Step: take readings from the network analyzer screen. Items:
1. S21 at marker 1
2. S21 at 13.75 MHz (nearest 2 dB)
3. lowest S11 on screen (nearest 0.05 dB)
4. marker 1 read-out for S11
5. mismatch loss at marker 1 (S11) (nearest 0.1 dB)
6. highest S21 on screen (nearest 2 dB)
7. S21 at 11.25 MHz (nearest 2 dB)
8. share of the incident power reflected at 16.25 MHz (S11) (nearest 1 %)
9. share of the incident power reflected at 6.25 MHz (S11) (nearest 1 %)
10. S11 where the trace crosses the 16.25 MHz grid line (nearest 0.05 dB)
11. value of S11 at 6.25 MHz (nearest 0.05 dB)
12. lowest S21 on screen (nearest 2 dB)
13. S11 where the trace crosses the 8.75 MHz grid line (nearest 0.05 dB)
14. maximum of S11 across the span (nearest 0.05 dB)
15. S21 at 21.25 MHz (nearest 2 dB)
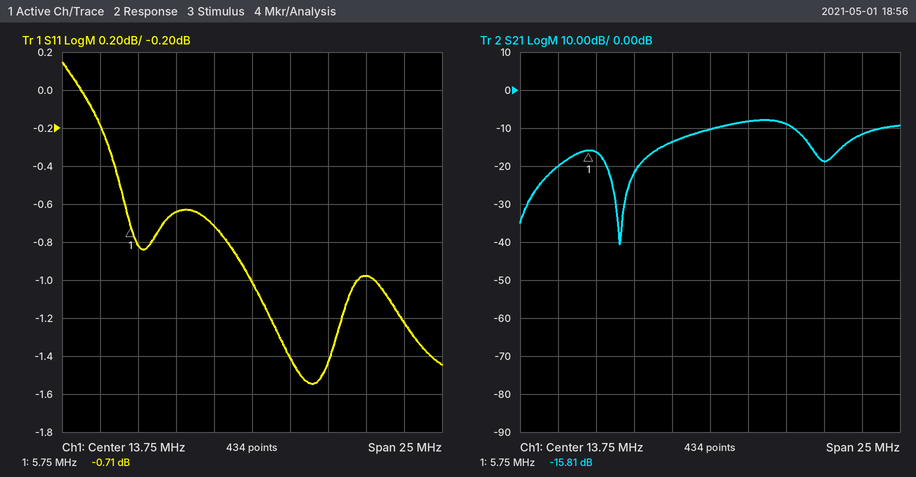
-15.81 dB
-10 dB
-1.55 dB
-0.71 dB
8.2 dB
-8 dB
-14 dB
72 %
83 %
-1.40 dB
-0.80 dB
-40 dB
-0.65 dB
0.15 dB
-18 dB
